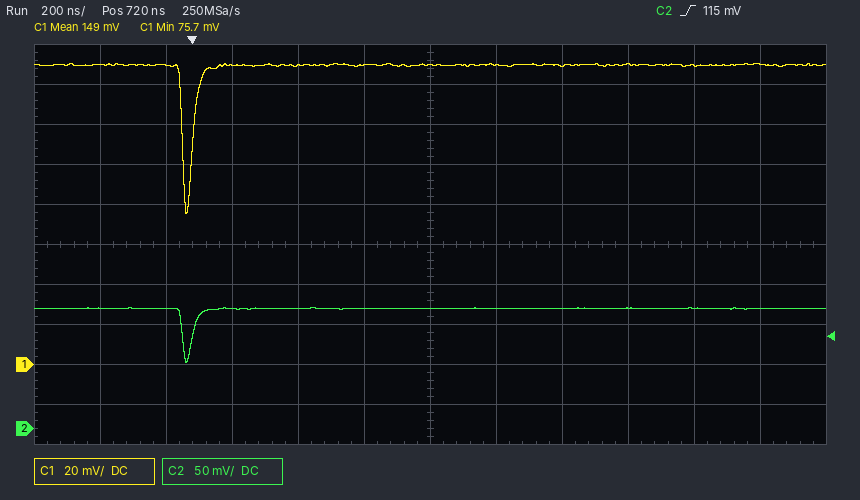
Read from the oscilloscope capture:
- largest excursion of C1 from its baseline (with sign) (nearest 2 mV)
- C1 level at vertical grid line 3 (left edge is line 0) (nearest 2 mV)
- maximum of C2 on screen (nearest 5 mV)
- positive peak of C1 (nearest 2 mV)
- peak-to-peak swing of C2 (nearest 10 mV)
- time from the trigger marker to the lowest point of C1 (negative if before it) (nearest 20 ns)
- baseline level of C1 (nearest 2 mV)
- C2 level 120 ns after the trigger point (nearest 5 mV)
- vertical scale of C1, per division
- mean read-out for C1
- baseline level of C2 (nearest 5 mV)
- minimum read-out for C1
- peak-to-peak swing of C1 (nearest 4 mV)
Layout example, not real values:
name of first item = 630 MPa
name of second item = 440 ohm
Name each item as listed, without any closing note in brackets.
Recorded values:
largest excursion of C1 from its baseline (with sign) = -74 mV
C1 level at vertical grid line 3 (left edge is line 0) = 150 mV
maximum of C2 on screen = 150 mV
positive peak of C1 = 150 mV
peak-to-peak swing of C2 = 70 mV
time from the trigger marker to the lowest point of C1 (negative if before it) = -20 ns
baseline level of C1 = 150 mV
C2 level 120 ns after the trigger point = 150 mV
vertical scale of C1, per division = 20 mV
mean read-out for C1 = 149 mV
baseline level of C2 = 150 mV
minimum read-out for C1 = 75.7 mV
peak-to-peak swing of C1 = 76 mV
